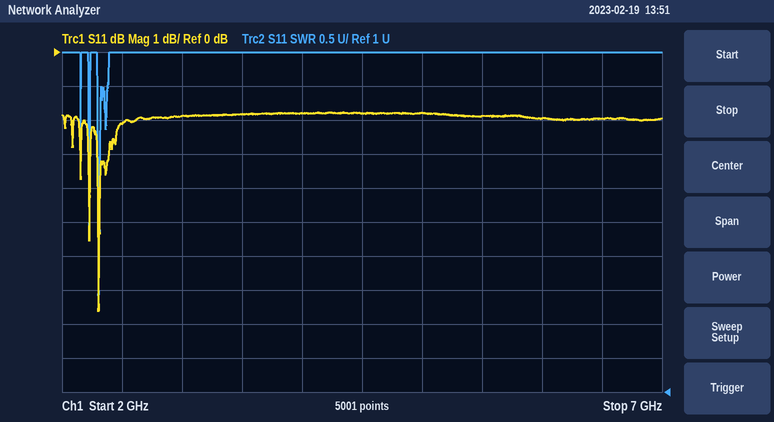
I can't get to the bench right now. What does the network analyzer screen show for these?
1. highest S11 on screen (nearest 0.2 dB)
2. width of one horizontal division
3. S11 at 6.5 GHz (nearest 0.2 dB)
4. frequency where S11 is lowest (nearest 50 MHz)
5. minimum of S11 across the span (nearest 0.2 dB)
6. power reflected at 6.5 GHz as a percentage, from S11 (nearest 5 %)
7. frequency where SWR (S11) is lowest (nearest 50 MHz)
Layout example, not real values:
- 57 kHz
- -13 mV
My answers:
- -1.8 dB
- 500 MHz
- -2.0 dB
- 2.30 GHz
- -7.6 dB
- 65 %
- 2.30 GHz
